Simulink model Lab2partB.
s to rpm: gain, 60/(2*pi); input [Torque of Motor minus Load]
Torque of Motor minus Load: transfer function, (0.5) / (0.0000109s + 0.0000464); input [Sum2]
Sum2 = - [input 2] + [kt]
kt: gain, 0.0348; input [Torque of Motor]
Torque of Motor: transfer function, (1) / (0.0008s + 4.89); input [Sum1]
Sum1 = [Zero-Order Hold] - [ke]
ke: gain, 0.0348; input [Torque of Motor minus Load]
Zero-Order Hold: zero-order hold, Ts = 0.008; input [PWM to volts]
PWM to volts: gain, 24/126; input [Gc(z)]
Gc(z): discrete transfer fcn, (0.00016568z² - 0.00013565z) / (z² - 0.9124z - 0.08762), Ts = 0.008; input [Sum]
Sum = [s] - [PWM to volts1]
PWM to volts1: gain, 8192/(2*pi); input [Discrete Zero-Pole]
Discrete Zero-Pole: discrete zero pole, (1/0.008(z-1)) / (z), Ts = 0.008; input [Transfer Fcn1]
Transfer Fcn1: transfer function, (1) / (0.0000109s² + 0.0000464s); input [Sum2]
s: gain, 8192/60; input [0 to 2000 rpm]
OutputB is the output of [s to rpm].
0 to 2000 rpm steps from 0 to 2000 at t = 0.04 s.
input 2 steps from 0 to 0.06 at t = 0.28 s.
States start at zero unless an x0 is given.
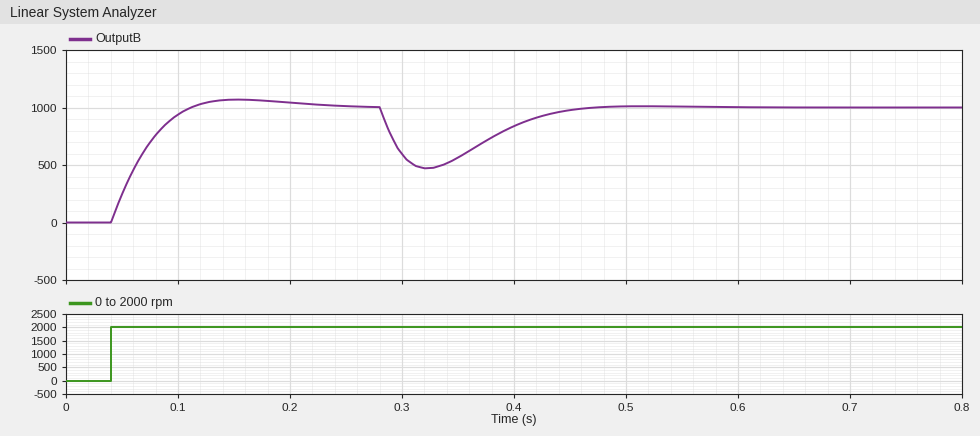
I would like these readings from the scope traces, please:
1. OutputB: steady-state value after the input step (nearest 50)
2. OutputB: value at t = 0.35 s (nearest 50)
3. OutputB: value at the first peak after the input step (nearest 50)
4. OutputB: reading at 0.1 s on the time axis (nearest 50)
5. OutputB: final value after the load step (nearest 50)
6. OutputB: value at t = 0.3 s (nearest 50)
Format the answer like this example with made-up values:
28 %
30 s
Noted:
1000
550
1050
950
1000
600
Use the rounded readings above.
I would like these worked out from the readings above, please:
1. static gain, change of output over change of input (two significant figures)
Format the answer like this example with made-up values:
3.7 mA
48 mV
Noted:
0.50
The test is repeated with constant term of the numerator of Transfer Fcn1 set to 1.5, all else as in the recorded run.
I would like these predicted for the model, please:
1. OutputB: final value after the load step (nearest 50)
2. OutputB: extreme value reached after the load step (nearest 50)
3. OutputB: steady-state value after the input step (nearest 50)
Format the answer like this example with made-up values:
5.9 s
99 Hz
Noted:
650
250
650
